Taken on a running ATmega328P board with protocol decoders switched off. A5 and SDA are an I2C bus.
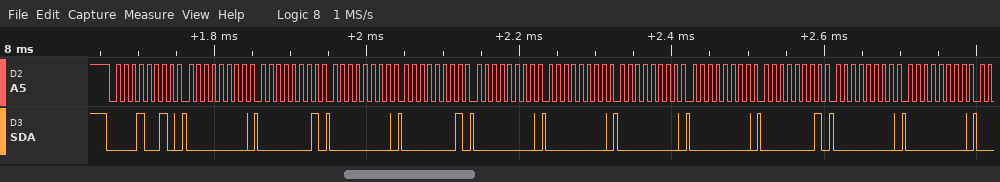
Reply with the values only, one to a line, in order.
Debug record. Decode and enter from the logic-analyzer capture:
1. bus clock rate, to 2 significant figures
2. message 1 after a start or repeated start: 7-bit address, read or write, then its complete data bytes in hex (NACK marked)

100 kHz
0x09 write: 00 01 00 01 00 00 00 00 01 00 00
